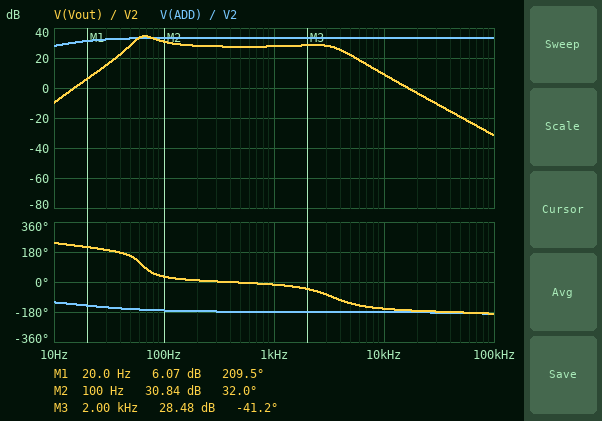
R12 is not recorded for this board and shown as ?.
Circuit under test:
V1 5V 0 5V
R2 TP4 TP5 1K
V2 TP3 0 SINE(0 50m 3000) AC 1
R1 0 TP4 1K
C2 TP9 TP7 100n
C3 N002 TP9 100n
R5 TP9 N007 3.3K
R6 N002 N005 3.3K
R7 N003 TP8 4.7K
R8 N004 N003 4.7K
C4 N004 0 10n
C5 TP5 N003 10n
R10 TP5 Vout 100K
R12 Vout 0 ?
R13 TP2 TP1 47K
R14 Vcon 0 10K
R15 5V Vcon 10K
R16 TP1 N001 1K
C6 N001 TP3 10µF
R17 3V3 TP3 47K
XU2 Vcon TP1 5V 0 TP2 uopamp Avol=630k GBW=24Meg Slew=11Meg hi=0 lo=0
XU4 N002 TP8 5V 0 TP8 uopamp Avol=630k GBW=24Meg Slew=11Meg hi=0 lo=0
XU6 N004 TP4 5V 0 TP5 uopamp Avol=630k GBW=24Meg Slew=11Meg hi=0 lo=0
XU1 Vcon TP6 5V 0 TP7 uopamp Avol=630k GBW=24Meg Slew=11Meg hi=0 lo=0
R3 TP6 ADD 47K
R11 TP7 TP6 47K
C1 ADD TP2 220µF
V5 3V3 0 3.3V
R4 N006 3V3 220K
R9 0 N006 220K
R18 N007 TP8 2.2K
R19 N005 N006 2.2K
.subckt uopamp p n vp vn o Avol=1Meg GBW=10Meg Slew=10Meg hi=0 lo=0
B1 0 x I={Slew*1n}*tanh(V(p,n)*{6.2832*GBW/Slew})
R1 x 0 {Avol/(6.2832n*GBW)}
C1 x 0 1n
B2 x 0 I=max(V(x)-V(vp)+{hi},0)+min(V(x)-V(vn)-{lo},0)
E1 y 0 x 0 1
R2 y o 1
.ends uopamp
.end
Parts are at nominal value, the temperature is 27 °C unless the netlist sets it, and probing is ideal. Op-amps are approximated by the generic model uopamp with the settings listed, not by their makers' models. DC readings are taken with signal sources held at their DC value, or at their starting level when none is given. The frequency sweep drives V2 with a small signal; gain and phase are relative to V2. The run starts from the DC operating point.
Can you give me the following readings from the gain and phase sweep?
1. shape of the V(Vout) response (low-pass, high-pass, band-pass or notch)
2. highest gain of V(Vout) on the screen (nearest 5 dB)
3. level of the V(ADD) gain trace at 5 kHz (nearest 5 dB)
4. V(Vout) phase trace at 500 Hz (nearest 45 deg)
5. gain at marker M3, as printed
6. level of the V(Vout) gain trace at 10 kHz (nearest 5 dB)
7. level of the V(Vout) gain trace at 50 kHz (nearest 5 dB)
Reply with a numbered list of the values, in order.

1. band-pass
2. 35 dB
3. 35 dB
4. 0 deg
5. 28.48 dB
6. 10 dB
7. -20 dB
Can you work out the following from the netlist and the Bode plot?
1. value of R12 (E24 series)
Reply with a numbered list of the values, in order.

1. 33 kΩ
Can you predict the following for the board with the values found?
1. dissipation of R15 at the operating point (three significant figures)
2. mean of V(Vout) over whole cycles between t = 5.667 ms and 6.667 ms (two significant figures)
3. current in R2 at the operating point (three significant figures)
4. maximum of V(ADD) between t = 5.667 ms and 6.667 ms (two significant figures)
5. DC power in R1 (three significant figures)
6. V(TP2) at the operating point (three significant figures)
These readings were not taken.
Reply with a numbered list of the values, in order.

1. 625 µW
2. 810 mV
3. 1.65 mA
4. 4.9 V
5. 2.72 mW
6. 2.50 V
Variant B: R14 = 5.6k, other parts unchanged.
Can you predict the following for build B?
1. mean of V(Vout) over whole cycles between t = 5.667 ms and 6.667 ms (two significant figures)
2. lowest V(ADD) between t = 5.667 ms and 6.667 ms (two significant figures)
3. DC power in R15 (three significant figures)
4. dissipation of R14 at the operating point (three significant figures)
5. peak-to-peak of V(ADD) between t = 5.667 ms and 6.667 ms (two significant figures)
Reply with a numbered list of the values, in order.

1. 770 mV
2. -1.8 mV
3. 1.03 mW
4. 575 µW
5. 4.1 V
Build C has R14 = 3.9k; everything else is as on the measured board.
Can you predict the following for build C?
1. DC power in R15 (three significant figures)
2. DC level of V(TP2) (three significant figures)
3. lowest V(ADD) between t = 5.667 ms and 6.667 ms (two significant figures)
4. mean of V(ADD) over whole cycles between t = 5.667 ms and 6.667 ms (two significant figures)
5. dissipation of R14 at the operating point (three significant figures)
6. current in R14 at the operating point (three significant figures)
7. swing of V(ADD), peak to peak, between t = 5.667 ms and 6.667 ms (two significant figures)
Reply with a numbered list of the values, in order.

1. 1.29 mW
2. 1.40 V
3. -3.1 mV
4. 1.5 V
5. 505 µW
6. 360 µA
7. 3.7 V
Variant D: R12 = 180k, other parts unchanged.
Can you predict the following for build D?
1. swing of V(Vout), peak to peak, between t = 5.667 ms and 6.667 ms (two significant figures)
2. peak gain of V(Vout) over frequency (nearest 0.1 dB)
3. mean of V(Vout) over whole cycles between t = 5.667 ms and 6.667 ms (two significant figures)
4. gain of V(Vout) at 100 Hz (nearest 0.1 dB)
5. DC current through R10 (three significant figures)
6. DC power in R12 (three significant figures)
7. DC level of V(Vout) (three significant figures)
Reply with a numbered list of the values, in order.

1. 3.2 V
2. 42.8 dB
3. 2.1 V
4. 39.1 dB
5. 11.8 µA
6. 25.0 µW
7. 2.12 V
